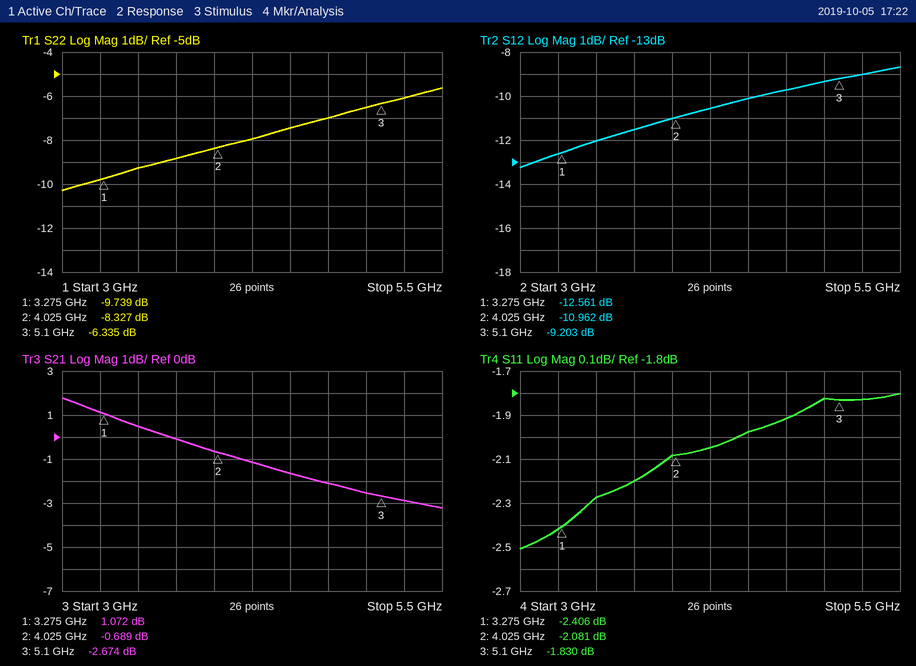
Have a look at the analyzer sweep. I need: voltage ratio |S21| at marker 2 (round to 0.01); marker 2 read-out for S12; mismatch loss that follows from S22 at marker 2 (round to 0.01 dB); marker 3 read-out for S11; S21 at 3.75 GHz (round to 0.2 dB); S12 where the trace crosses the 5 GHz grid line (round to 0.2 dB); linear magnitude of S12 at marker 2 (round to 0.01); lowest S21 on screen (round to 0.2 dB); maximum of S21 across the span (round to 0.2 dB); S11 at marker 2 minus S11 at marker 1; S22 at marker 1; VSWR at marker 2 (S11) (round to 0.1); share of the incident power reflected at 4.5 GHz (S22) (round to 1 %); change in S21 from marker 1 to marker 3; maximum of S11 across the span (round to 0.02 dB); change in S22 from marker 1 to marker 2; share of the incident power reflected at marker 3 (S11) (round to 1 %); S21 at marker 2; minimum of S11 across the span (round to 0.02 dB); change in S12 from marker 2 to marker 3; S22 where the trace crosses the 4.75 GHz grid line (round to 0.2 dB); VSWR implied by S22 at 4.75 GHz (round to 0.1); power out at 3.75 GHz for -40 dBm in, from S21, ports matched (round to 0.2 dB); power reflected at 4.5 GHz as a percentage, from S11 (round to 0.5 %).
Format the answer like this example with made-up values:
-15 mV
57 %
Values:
0.92
-10.962 dB
0.69 dB
-1.830 dB
0.0 dB
-9.4 dB
0.28
-3.2 dB
1.8 dB
0.325 dB
-9.739 dB
8.4
18 %
-3.746 dB
-1.80 dB
1.412 dB
66 %
-0.689 dB
-2.50 dB
1.759 dB
-7.0 dB
2.6
-40.0 dBm
63.5 %
